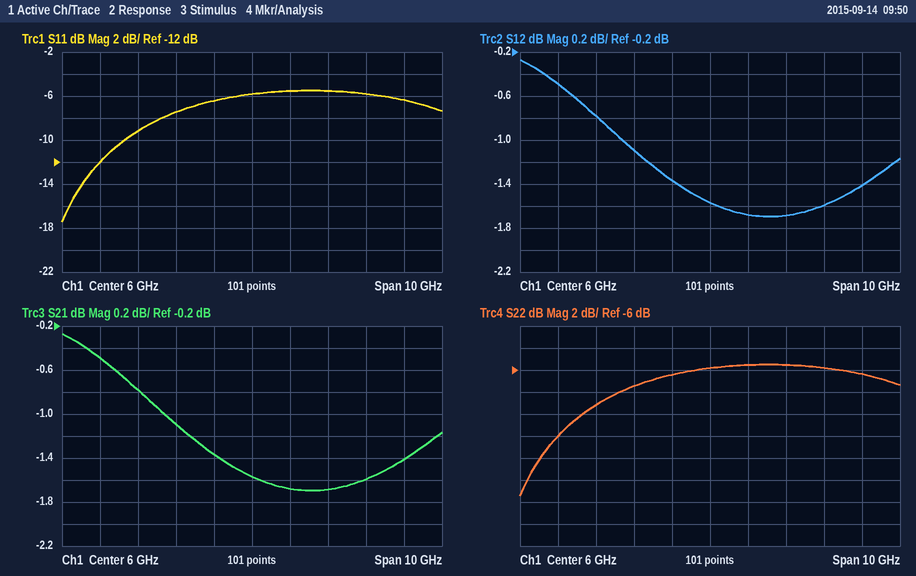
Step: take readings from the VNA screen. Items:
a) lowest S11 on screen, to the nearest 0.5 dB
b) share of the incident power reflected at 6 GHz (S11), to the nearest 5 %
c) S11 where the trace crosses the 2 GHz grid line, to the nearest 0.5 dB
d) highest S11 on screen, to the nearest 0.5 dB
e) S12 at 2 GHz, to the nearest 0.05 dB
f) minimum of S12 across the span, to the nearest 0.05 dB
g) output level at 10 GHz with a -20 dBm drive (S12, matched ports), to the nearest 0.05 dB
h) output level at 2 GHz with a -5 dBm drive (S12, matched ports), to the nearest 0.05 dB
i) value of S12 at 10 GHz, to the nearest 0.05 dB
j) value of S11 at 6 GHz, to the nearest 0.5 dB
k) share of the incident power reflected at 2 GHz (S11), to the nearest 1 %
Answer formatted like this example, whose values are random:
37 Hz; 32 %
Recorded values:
-17.5 dB; 25 %; -12.0 dB; -5.5 dB; -0.50 dB; -1.70 dB; -21.40 dBm; -5.50 dBm; -1.40 dB; -6.0 dB; 6 %
